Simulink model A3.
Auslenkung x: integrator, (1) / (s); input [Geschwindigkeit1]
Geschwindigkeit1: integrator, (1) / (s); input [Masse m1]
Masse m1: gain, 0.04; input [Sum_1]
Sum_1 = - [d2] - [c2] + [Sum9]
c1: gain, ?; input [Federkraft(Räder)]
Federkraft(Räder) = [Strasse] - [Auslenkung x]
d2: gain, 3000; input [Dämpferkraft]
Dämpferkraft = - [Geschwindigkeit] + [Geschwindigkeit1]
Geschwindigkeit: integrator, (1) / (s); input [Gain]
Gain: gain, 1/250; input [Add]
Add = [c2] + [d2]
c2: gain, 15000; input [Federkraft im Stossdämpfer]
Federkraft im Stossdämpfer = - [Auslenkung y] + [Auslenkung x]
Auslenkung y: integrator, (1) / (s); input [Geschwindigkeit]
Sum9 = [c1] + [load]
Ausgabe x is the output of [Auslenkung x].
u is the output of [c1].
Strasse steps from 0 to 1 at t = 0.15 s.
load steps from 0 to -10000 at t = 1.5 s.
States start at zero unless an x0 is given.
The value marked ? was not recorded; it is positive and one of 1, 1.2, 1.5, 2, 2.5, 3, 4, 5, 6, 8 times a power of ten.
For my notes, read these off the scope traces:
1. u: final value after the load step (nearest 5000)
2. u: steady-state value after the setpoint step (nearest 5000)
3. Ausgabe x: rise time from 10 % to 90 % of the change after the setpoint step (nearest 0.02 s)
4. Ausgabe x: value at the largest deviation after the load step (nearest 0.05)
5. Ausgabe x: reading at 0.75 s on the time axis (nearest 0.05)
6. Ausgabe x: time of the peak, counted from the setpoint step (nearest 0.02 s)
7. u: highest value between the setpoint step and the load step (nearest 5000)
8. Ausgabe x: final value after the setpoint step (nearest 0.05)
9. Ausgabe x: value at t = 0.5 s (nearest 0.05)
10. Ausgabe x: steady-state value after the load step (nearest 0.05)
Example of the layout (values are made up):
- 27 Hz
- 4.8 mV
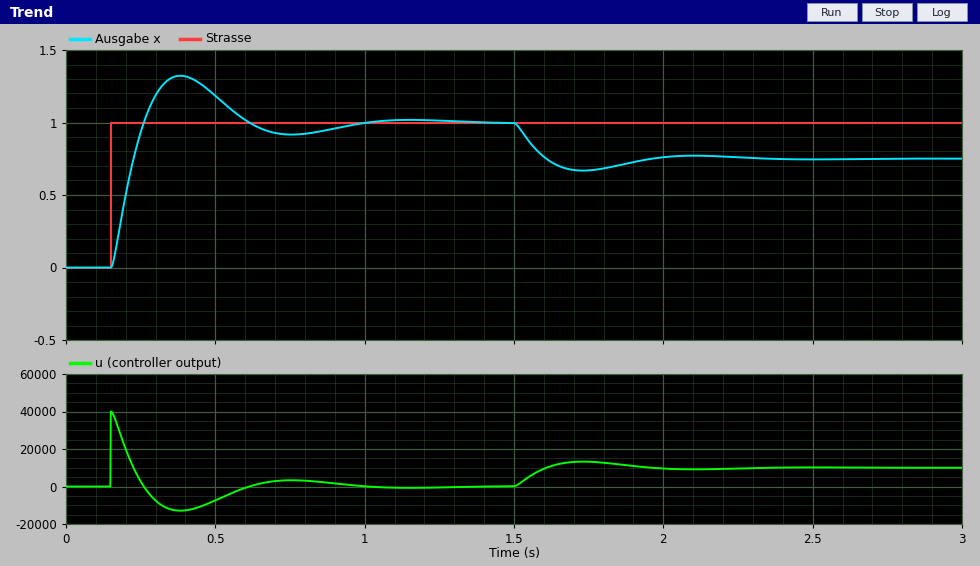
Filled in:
- 10000
- 0
- 0.08 s
- 0.65
- 0.90
- 0.24 s
- 40000
- 1.00
- 1.20
- 0.75
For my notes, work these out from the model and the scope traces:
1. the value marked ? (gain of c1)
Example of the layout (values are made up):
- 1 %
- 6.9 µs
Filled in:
- 40000
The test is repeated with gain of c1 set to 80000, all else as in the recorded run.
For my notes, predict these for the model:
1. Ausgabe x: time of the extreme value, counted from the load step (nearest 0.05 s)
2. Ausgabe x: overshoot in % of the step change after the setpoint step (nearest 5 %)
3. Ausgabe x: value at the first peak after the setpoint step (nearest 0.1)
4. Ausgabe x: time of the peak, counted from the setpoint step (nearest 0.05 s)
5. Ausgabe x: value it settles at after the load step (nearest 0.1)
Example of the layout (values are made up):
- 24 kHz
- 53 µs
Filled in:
- 0.15 s
- 20 %
- 1.2
- 0.15 s
- 0.9
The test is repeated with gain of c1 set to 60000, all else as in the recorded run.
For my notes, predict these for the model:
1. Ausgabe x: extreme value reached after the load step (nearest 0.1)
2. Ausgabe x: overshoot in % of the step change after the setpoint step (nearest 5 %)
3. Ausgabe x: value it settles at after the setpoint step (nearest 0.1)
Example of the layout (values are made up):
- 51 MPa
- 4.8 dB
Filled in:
- 0.8
- 25 %
- 1.0
